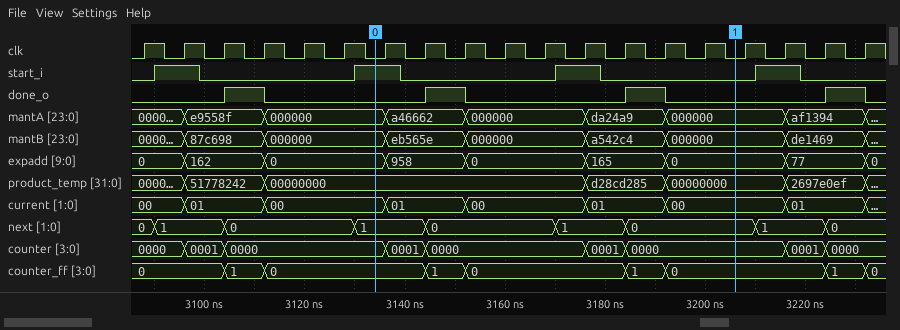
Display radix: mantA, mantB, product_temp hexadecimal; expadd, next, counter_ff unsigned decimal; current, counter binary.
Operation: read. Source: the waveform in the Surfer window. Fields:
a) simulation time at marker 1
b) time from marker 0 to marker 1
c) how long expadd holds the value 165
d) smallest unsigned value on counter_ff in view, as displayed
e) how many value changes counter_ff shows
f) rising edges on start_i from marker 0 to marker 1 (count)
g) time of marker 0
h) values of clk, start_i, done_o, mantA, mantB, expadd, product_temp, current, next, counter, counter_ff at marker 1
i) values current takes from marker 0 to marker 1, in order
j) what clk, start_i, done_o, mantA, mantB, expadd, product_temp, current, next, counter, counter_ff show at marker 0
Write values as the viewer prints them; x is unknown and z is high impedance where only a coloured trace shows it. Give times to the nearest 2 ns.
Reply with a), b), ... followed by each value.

a) 3206 ns
b) 72 ns
c) 16 ns
d) 0
e) 8
f) 1
g) 3134 ns
h) clk=0, start_i=0, done_o=0, mantA=000000, mantB=000000, expadd=0, product_temp=00000000, current=00, next=0, counter=0000, counter_ff=0
i) 00, 01, 00, 01, 00
j) clk=0, start_i=1, done_o=0, mantA=000000, mantB=000000, expadd=0, product_temp=00000000, current=00, next=1, counter=0000, counter_ff=0
